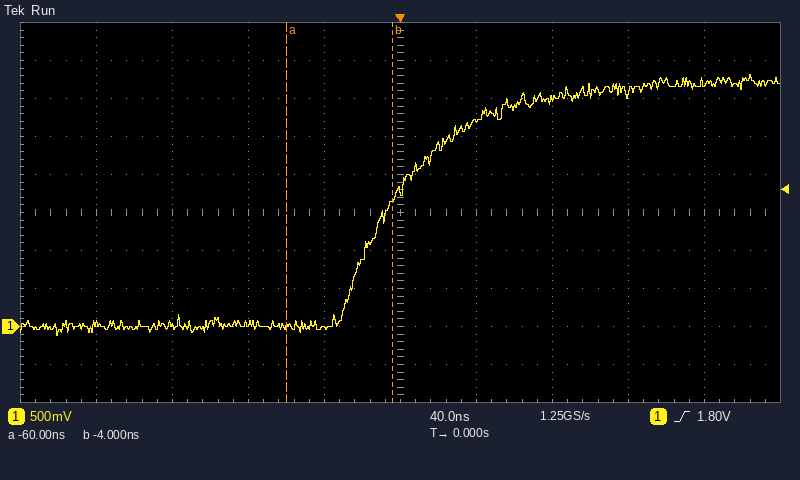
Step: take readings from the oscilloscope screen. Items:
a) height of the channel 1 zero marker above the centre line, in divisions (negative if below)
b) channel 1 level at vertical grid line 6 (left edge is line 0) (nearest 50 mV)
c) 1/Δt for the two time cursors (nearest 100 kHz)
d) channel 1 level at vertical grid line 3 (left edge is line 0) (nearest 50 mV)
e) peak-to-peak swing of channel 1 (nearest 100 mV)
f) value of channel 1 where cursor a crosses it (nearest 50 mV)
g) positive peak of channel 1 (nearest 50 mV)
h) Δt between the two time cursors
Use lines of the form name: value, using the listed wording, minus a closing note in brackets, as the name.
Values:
height of the channel 1 zero marker above the centre line, in divisions: -3.0 div
channel 1 level at vertical grid line 6 (left edge is line 0): 2.70 V
1/Δt for the two time cursors: 17.9 MHz
channel 1 level at vertical grid line 3 (left edge is line 0): 50 mV
peak-to-peak swing of channel 1: 3.40 V
value of channel 1 where cursor a crosses it: 0 mV
positive peak of channel 1: 3.30 V
Δt between the two time cursors: 56 ns
